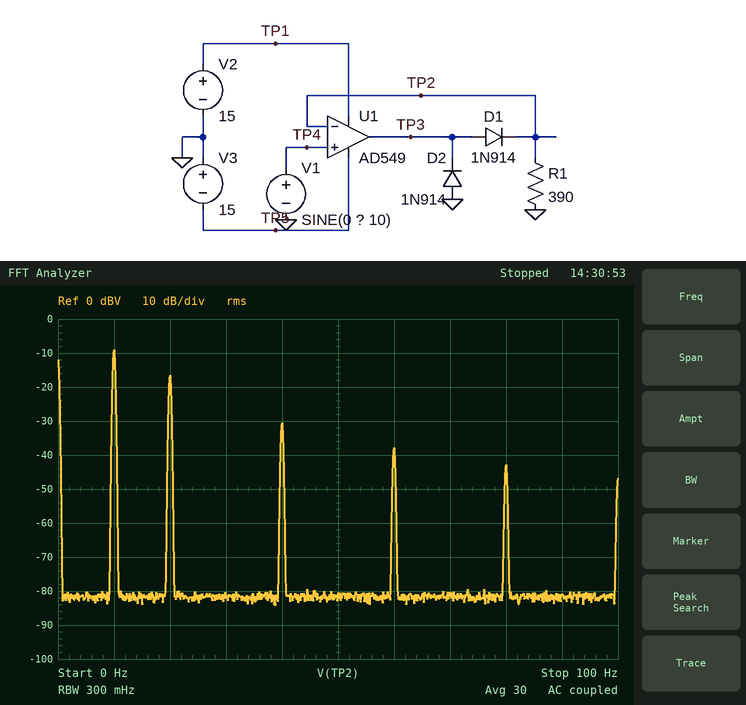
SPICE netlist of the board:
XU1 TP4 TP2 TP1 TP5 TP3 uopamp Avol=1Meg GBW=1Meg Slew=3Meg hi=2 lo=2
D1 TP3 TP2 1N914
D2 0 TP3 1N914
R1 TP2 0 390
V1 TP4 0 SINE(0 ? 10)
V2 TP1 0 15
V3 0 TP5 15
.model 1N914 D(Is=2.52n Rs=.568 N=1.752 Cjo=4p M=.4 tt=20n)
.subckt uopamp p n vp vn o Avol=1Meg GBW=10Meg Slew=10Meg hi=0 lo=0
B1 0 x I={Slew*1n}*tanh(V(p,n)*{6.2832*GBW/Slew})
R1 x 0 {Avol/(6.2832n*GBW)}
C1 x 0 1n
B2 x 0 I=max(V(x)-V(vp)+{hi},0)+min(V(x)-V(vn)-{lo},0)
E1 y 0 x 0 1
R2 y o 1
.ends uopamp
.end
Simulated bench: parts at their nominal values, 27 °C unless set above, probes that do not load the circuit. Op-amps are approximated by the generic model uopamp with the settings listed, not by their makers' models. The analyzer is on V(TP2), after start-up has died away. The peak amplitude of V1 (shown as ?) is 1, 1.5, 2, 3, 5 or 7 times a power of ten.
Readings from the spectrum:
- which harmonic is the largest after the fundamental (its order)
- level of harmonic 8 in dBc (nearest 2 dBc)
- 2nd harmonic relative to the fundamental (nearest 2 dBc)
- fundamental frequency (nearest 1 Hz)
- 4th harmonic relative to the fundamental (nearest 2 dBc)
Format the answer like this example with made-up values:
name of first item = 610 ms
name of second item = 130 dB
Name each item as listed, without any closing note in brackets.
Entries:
which harmonic is the largest after the fundamental = 2
level of harmonic 8 in dBc = -34 dBc
2nd harmonic relative to the fundamental = -8 dBc
fundamental frequency = 10 Hz
4th harmonic relative to the fundamental = -22 dBc
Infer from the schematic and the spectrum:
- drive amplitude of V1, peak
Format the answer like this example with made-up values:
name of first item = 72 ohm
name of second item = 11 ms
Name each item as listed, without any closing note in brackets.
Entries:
drive amplitude of V1, peak = 1 V
